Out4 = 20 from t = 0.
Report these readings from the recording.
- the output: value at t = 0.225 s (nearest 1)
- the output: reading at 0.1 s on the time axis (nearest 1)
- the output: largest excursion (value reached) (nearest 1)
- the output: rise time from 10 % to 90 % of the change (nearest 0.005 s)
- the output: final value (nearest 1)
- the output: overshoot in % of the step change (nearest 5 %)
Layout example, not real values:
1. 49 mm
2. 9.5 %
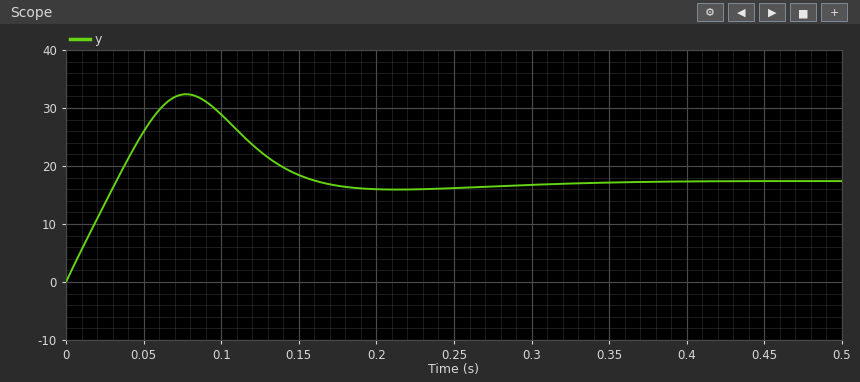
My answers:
1. 16
2. 29
3. 32
4. 0.025 s
5. 17
6. 85 %
